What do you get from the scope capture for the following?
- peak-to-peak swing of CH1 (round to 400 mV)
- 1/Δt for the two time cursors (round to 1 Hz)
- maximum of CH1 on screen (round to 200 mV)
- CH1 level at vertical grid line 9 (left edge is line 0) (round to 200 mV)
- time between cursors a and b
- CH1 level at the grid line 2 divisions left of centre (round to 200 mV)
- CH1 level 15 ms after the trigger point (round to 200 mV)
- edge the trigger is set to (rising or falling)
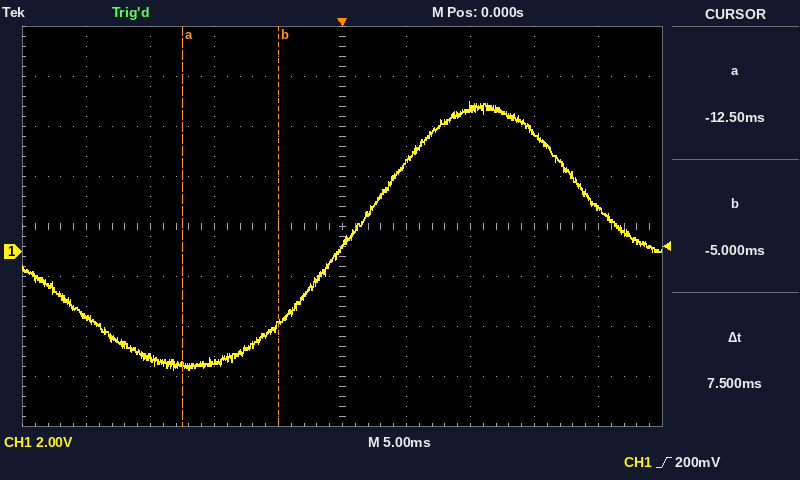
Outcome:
10.8 V
133 Hz
6.0 V
1.8 V
7.5 ms
-4.4 V
4.8 V
rising
